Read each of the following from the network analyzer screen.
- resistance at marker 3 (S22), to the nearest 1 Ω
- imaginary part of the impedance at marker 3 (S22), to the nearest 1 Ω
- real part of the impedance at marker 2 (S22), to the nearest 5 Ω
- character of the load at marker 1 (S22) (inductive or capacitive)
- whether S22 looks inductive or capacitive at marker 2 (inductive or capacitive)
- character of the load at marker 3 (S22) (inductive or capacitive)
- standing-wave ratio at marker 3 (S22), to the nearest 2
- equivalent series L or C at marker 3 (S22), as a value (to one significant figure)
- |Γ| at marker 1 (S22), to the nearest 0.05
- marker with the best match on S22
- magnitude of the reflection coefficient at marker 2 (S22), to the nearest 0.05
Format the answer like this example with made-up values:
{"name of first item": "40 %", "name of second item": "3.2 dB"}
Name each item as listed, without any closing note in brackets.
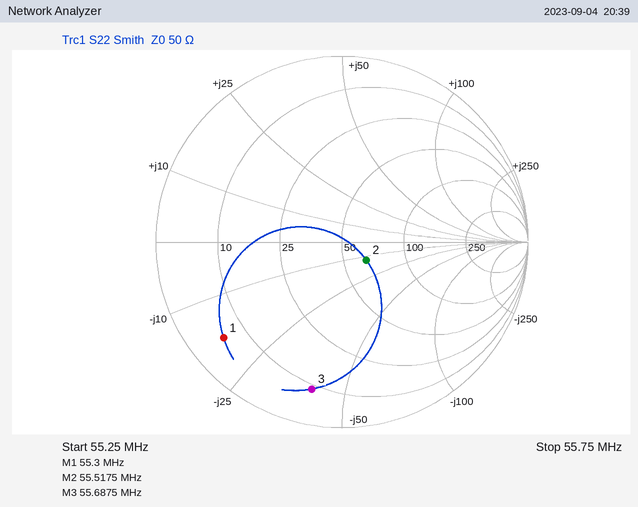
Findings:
{"resistance at marker 3 (S22), to the nearest 1 Ω": "9 Ω", "imaginary part of the impedance at marker 3 (S22), to the nearest 1 Ω": "-40 Ω", "real part of the impedance at marker 2 (S22), to the nearest 5 Ω": "65 Ω", "character of the load at marker 1 (S22)": "capacitive", "whether S22 looks inductive or capacitive at marker 2": "capacitive", "character of the load at marker 3 (S22)": "capacitive", "standing-wave ratio at marker 3 (S22), to the nearest 2": "10", "equivalent series L or C at marker 3 (S22), as a value": "70 pF", "|Γ| at marker 1 (S22), to the nearest 0.05": "0.80", "marker with the best match on S22": "marker 2", "magnitude of the reflection coefficient at marker 2 (S22), to the nearest 0.05": "0.15"}
